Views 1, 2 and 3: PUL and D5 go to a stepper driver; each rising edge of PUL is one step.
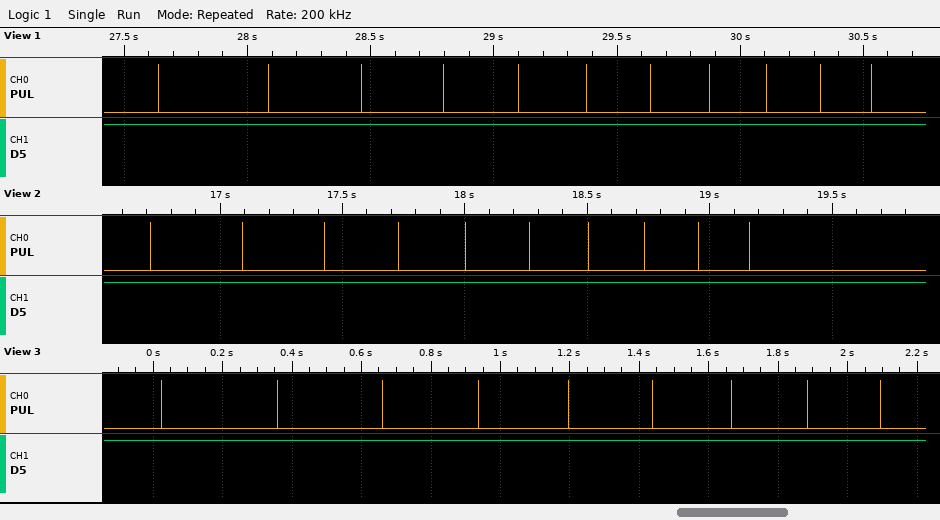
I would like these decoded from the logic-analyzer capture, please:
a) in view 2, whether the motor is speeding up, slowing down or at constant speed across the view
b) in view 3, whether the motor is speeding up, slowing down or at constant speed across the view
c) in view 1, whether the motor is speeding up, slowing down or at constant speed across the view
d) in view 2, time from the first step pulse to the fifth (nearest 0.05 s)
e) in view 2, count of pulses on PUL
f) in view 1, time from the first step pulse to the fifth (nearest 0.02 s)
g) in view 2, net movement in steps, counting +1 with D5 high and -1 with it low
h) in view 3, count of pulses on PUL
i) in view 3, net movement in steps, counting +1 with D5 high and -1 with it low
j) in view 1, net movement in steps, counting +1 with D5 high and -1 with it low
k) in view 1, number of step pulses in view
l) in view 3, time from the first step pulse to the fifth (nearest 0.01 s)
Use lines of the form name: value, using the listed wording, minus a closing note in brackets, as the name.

in view 2, whether the motor is speeding up, slowing down or at constant speed across the view: speeding up
in view 3, whether the motor is speeding up, slowing down or at constant speed across the view: speeding up
in view 1, whether the motor is speeding up, slowing down or at constant speed across the view: speeding up
in view 2, time from the first step pulse to the fifth: 1.30 s
in view 2, count of pulses on PUL: 10
in view 1, time from the first step pulse to the fifth: 1.46 s
in view 2, net movement in steps, counting +1 with D5 high and -1 with it low: +10
in view 3, count of pulses on PUL: 9
in view 3, net movement in steps, counting +1 with D5 high and -1 with it low: +9
in view 1, net movement in steps, counting +1 with D5 high and -1 with it low: +11
in view 1, number of step pulses in view: 11
in view 3, time from the first step pulse to the fifth: 1.17 s
